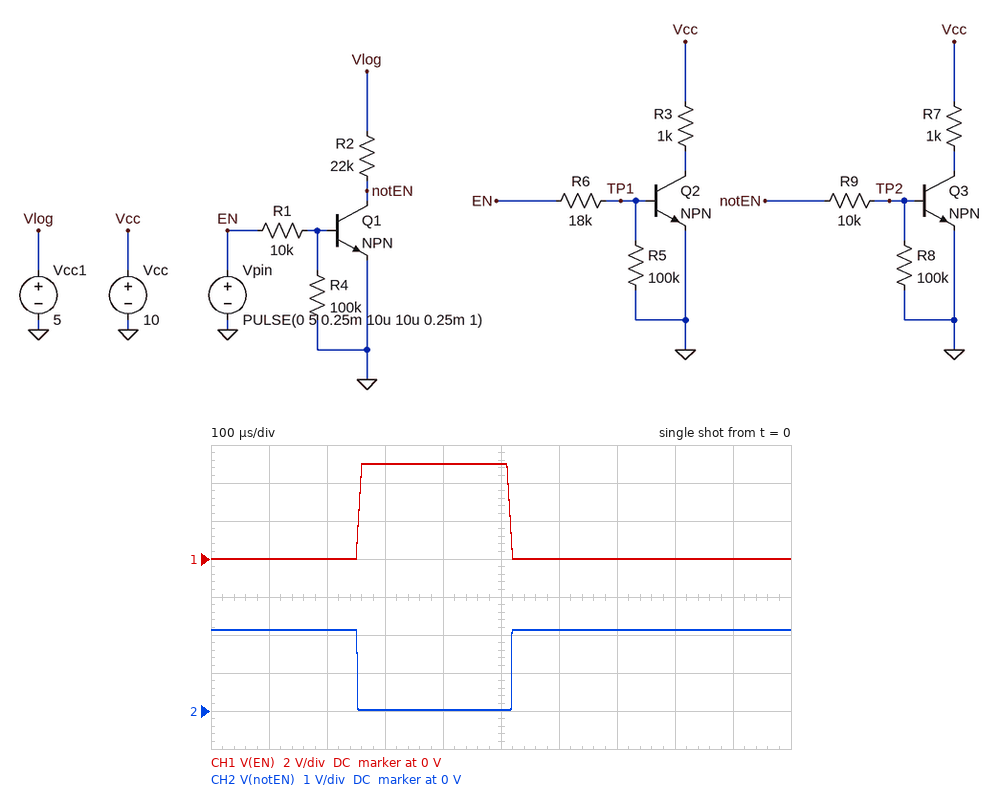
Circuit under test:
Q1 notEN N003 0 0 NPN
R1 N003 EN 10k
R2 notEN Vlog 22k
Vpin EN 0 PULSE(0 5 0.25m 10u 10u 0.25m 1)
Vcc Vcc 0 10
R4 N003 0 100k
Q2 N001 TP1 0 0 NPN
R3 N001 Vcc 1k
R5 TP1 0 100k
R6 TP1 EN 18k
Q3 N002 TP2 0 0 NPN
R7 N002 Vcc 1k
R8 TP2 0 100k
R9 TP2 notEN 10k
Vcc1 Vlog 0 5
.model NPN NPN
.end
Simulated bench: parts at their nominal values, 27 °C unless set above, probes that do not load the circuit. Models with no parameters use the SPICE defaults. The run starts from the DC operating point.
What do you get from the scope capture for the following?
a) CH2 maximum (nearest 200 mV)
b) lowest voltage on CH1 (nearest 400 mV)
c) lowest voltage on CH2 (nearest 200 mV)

2.2 V
0 V
0 V
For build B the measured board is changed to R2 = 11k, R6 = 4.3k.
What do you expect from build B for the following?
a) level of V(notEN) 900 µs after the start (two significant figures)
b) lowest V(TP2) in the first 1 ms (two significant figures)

2.8 V
27 mV
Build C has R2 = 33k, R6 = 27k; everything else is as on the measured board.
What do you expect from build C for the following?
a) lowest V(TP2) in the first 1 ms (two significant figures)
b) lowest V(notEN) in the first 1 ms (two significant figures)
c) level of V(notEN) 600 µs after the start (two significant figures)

20 mV
22 mV
1.8 V
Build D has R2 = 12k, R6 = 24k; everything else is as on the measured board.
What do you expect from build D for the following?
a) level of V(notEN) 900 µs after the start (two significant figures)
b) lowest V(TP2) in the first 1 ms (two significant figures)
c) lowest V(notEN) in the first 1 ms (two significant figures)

2.7 V
26 mV
29 mV
